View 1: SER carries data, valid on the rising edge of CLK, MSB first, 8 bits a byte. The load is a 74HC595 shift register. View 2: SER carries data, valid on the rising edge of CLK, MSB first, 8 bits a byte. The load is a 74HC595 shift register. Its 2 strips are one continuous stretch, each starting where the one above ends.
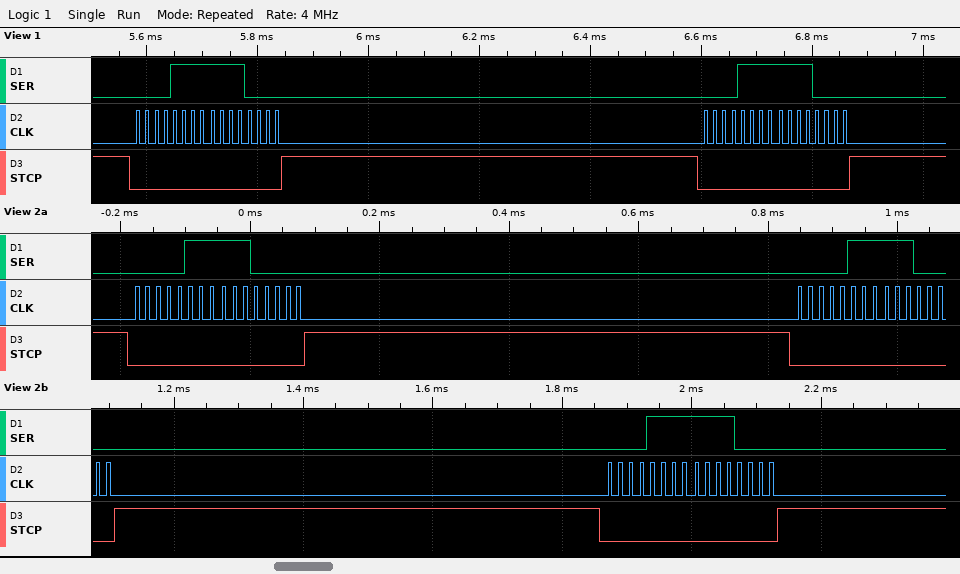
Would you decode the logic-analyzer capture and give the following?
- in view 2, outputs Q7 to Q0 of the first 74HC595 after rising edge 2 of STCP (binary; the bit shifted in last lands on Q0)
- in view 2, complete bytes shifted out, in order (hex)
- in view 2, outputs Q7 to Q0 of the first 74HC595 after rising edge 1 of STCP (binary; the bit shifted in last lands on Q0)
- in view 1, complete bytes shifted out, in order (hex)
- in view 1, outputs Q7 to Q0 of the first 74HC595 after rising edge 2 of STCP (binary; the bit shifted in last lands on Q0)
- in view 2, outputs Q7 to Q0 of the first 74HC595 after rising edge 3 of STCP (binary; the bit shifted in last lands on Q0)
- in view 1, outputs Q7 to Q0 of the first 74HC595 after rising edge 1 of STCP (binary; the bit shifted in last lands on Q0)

11100000
07 E0 07 E0 0F F0
11100000
0F F0 0F F0
11110000
11110000
11110000
